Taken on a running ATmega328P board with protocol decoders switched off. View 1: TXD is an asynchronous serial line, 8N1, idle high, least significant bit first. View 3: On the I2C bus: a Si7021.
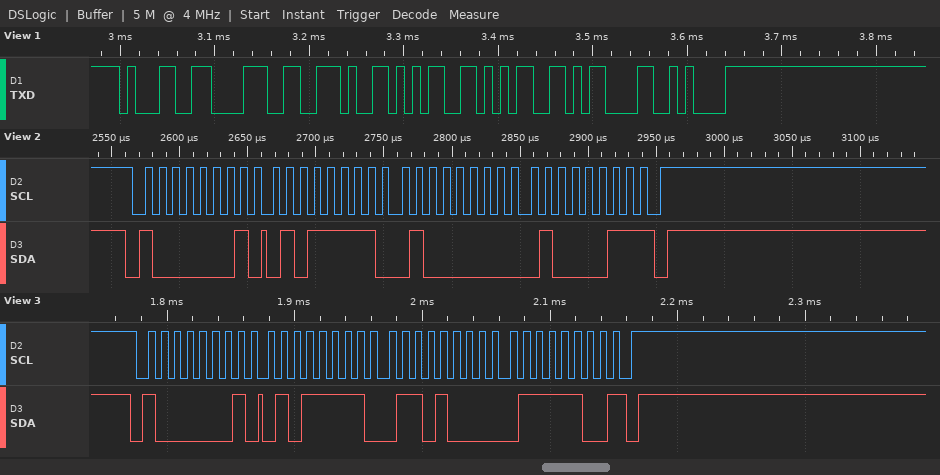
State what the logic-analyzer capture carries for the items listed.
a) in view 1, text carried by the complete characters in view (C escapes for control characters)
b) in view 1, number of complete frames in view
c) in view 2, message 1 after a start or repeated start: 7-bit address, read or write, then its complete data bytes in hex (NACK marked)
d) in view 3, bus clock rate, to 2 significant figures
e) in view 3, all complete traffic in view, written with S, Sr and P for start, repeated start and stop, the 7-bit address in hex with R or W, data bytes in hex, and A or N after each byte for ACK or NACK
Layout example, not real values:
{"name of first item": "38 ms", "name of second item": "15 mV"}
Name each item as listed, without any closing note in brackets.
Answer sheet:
{"in view 1, text carried by the complete characters in view": "\"18.55\\r\\n\"", "in view 1, number of complete frames in view": "7", "in view 2, message 1 after a start or repeated start: 7-bit address, read or write, then its complete data bytes in hex": "0x40 read: 5F 40 43 NACK", "in view 3, bus clock rate, to 2 significant figures": "100 kHz", "in view 3, all complete traffic in view, written with S, Sr and P for start, repeated start and stop, the 7-bit address in hex with R or W, data bytes in hex, and A or N after each byte for ACK or NACK": "S 40R A 5F A 68 A 7C N P"}
